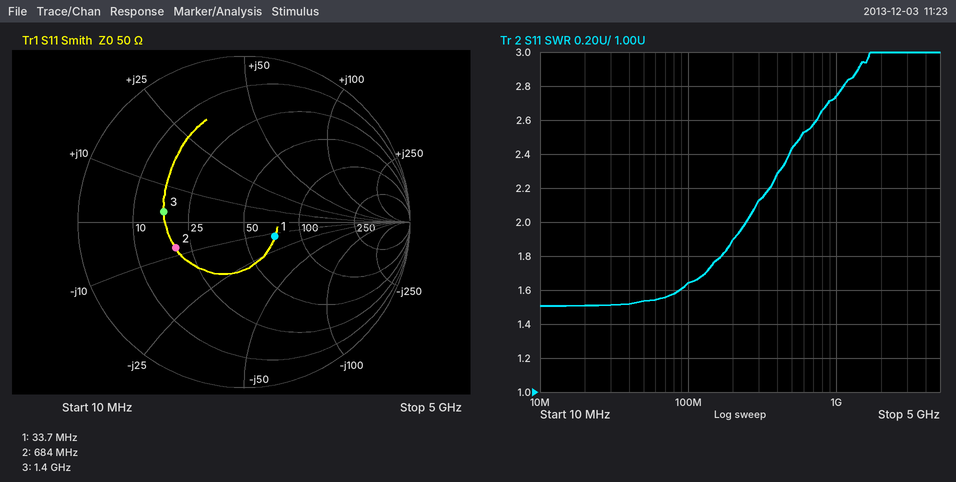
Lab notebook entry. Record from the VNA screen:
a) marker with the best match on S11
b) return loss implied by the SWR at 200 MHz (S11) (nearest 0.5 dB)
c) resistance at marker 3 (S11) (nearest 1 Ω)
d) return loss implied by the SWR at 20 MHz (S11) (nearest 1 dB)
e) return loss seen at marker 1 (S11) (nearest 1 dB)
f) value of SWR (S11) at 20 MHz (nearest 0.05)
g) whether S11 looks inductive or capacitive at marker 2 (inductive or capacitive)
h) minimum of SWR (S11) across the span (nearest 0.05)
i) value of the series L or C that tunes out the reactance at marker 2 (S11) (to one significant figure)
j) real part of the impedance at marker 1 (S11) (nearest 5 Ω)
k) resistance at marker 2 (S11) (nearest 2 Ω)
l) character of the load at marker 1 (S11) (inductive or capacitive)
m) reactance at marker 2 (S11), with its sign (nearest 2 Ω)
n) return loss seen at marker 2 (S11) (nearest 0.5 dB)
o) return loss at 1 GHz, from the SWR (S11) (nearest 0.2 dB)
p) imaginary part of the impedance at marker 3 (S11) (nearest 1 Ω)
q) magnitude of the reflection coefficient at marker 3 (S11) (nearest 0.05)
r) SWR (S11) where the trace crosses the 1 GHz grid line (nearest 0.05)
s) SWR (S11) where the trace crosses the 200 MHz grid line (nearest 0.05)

marker 1
10.0 dB
17 Ω
14 dB
14 dB
1.50
capacitive
1.50
2 nH
70 Ω
20 Ω
capacitive
-8 Ω
7.0 dB
6.6 dB
+3 Ω
0.50
2.75
1.90
